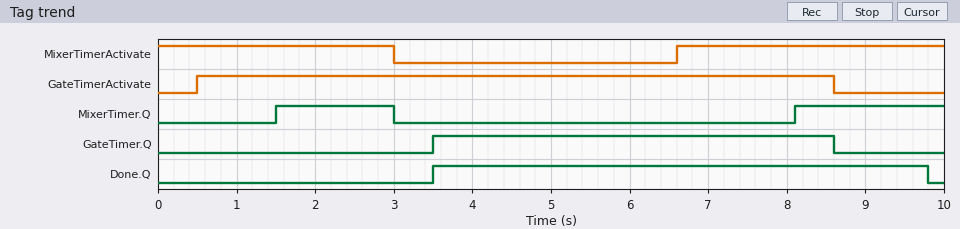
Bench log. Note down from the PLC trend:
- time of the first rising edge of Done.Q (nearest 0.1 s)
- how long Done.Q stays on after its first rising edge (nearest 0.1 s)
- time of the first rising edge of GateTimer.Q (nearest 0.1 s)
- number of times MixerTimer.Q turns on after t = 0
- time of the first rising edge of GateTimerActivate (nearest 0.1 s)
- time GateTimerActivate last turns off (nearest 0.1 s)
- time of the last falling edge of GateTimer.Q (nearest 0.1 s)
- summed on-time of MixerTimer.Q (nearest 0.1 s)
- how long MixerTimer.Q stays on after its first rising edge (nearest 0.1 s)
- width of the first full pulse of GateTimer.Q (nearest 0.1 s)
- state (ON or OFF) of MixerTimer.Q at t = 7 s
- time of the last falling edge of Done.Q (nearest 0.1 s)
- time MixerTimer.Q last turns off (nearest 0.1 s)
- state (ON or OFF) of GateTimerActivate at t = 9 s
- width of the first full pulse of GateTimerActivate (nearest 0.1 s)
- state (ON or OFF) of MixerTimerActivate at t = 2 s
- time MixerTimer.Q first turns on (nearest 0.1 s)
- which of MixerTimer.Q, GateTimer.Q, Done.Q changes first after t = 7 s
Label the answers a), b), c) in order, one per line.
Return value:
a) 3.5 s
b) 6.3 s
c) 3.5 s
d) 2
e) 0.5 s
f) 8.6 s
g) 8.6 s
h) 3.4 s
i) 1.5 s
j) 5.1 s
k) OFF
l) 9.8 s
m) 3.0 s
n) OFF
o) 8.1 s
p) ON
q) 1.5 s
r) MixerTimer.Q
